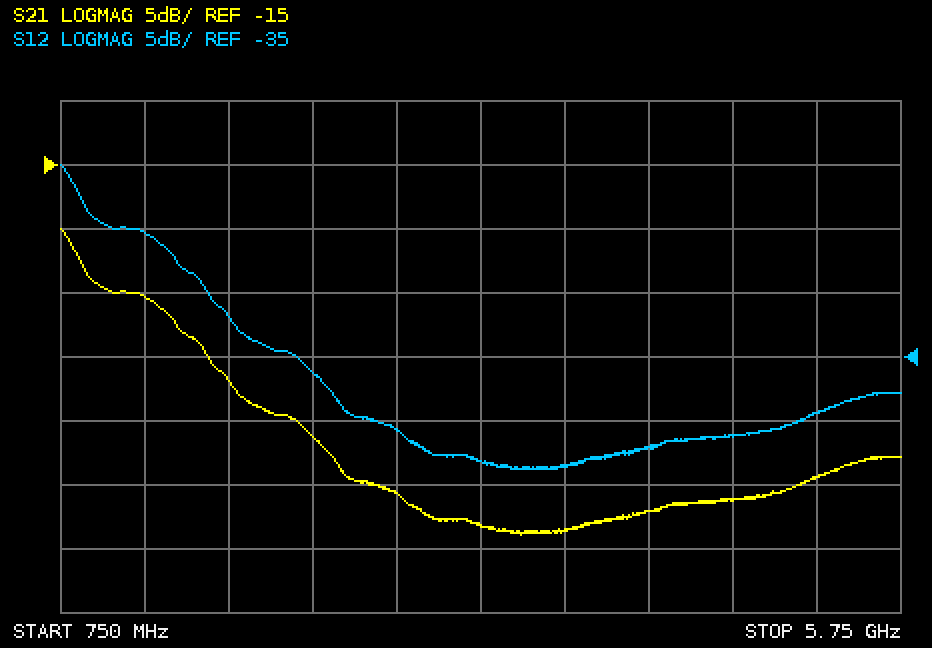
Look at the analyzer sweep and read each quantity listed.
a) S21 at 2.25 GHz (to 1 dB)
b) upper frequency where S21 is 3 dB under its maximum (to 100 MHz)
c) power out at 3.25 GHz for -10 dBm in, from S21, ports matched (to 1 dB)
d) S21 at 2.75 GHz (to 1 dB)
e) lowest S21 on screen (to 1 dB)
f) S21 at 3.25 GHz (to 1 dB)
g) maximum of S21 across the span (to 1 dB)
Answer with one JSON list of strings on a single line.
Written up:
["-36 dB", "900 MHz", "-53 dBm", "-41 dB", "-44 dB", "-43 dB", "-20 dB"]
